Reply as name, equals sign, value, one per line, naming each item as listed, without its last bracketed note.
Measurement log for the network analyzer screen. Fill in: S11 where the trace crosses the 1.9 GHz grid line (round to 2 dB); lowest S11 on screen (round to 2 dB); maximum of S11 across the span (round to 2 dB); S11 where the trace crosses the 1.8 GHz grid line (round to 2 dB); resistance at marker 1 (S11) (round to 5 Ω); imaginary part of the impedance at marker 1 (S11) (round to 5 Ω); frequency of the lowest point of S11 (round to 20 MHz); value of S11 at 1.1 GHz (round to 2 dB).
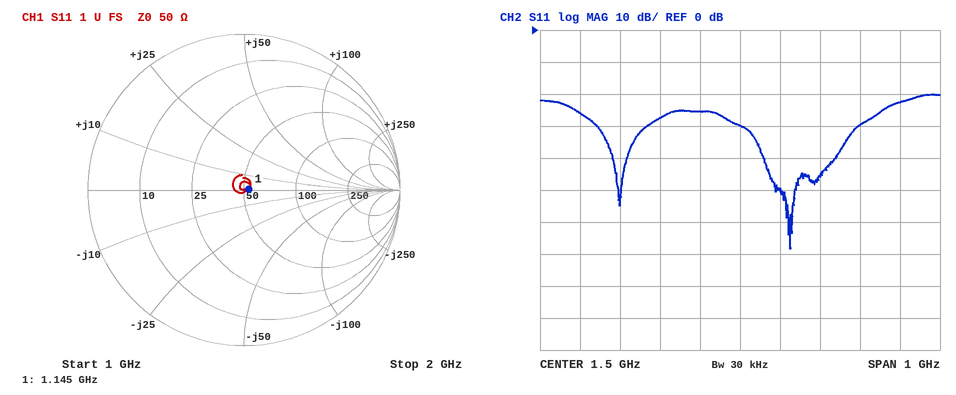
S11 where the trace crosses the 1.9 GHz grid line = -22 dB
lowest S11 on screen = -68 dB
maximum of S11 across the span = -20 dB
S11 where the trace crosses the 1.8 GHz grid line = -30 dB
resistance at marker 1 (S11) = 55 Ω
imaginary part of the impedance at marker 1 (S11) = 0 Ω
frequency of the lowest point of S11 = 1.62 GHz
value of S11 at 1.1 GHz = -26 dB
